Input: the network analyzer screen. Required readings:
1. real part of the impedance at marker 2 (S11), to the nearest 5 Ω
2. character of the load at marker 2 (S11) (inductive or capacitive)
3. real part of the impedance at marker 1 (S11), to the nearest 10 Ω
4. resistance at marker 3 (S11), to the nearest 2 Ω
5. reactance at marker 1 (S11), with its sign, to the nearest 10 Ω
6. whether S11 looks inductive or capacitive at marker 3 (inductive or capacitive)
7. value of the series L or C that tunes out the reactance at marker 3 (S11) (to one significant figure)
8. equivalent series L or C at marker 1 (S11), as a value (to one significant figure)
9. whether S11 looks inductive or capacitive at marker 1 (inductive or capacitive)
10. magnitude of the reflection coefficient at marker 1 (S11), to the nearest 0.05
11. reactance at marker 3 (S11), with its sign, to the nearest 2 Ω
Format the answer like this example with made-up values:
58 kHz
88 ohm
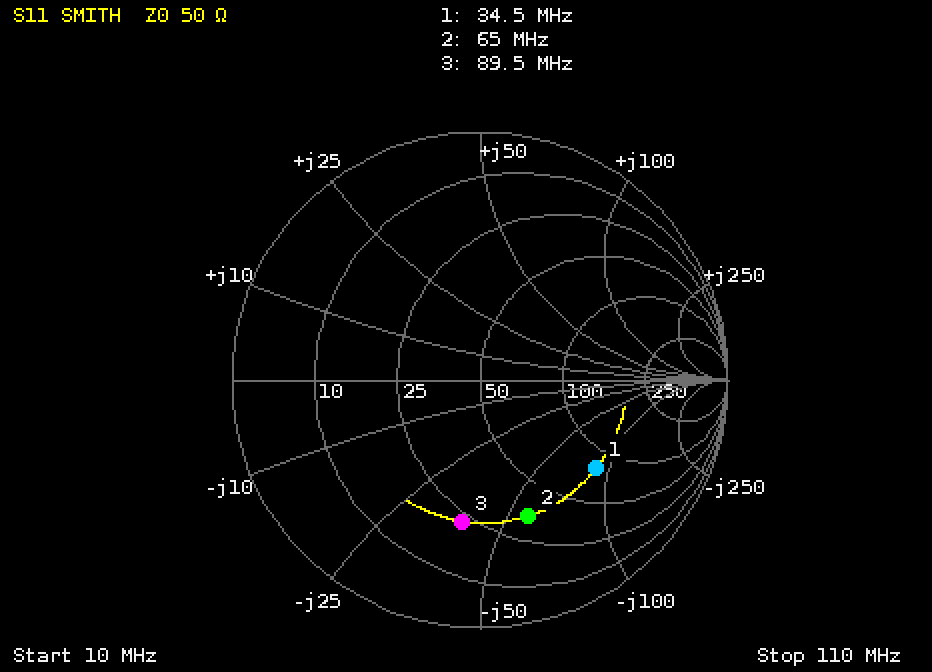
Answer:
35 Ω
capacitive
80 Ω
22 Ω
-90 Ω
capacitive
70 nH
50 pF
capacitive
0.60
-38 Ω
